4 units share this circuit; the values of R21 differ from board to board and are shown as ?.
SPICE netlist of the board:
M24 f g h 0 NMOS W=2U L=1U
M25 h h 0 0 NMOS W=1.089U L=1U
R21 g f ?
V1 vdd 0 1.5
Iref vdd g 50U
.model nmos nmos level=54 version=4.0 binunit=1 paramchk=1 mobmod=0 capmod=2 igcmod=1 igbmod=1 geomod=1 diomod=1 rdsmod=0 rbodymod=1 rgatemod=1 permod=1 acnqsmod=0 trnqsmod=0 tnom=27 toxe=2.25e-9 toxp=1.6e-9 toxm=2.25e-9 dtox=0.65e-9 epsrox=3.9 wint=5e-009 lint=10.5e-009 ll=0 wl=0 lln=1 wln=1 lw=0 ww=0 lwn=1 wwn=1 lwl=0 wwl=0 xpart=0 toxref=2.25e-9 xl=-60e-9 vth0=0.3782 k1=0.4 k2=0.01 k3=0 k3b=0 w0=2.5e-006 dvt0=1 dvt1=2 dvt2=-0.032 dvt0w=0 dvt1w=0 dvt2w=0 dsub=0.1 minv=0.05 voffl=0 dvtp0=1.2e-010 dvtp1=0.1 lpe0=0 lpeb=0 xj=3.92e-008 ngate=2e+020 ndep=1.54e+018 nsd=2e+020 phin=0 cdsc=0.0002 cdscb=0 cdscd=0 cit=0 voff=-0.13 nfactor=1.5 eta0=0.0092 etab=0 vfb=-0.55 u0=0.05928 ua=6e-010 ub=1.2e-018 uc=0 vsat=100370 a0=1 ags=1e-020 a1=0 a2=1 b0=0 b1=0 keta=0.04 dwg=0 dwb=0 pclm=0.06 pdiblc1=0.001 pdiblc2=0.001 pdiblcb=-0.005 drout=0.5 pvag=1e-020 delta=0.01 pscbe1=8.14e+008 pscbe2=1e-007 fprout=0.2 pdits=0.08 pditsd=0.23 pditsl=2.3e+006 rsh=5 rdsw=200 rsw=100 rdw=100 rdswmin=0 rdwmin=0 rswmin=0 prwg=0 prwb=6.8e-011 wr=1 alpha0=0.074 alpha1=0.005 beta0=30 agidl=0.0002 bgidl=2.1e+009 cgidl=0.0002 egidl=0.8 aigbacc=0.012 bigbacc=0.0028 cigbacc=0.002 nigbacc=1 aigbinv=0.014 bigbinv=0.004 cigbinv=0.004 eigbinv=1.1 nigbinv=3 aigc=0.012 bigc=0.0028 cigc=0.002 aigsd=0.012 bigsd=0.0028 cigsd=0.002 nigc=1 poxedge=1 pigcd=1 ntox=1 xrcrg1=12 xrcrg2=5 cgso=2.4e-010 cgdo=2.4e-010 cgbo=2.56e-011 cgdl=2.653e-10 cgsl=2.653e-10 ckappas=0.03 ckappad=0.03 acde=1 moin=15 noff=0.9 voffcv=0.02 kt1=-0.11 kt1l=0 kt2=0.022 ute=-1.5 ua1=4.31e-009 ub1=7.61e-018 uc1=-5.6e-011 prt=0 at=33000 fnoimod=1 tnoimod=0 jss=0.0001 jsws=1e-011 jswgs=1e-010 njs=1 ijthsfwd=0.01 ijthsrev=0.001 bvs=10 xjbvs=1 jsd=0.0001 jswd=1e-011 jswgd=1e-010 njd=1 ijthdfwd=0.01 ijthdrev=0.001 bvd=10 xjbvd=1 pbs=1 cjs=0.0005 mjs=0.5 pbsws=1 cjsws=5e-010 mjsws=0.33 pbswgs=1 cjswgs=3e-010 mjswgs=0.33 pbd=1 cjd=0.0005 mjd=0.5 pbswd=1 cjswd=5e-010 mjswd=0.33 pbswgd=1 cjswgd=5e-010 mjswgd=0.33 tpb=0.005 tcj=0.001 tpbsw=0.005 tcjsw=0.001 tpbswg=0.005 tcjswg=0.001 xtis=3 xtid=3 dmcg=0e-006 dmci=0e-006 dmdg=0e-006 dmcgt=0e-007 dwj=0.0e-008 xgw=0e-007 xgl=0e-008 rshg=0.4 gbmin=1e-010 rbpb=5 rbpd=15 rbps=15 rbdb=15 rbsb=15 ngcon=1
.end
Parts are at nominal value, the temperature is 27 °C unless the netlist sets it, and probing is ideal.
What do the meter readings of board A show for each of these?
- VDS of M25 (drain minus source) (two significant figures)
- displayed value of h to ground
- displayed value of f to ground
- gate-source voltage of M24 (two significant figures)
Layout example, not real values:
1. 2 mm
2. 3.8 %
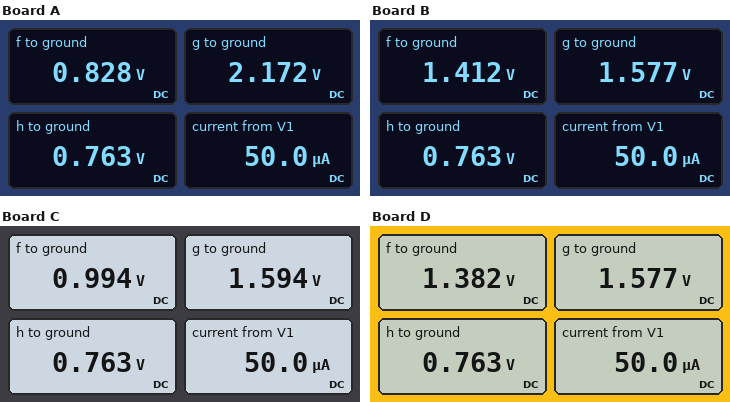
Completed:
1. 760 mV
2. 0.763 V
3. 0.828 V
4. 1.4 V
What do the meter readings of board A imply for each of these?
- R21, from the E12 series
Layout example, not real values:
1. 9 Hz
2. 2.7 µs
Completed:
1. 27 kΩ
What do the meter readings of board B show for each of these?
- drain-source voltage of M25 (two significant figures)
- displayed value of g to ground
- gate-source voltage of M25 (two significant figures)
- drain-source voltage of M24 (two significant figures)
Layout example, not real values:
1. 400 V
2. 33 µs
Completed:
1. 760 mV
2. 1.577 V
3. 760 mV
4. 650 mV
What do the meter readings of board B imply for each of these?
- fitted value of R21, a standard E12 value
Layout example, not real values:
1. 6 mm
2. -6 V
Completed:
1. 3.3 kΩ
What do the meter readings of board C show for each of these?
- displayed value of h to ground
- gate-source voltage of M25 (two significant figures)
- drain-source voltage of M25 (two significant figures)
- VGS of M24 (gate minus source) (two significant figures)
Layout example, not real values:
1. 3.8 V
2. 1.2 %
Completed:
1. 0.763 V
2. 760 mV
3. 760 mV
4. 830 mV
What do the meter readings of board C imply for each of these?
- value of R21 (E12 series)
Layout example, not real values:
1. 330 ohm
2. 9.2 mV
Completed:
1. 12 kΩ
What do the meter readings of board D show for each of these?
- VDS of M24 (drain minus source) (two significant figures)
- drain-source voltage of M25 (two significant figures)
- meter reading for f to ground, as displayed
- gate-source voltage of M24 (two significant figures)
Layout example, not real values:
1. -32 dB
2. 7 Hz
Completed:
1. 620 mV
2. 760 mV
3. 1.382 V
4. 810 mV
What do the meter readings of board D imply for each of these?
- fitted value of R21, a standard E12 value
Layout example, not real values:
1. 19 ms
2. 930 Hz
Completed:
1. 3.9 kΩ
